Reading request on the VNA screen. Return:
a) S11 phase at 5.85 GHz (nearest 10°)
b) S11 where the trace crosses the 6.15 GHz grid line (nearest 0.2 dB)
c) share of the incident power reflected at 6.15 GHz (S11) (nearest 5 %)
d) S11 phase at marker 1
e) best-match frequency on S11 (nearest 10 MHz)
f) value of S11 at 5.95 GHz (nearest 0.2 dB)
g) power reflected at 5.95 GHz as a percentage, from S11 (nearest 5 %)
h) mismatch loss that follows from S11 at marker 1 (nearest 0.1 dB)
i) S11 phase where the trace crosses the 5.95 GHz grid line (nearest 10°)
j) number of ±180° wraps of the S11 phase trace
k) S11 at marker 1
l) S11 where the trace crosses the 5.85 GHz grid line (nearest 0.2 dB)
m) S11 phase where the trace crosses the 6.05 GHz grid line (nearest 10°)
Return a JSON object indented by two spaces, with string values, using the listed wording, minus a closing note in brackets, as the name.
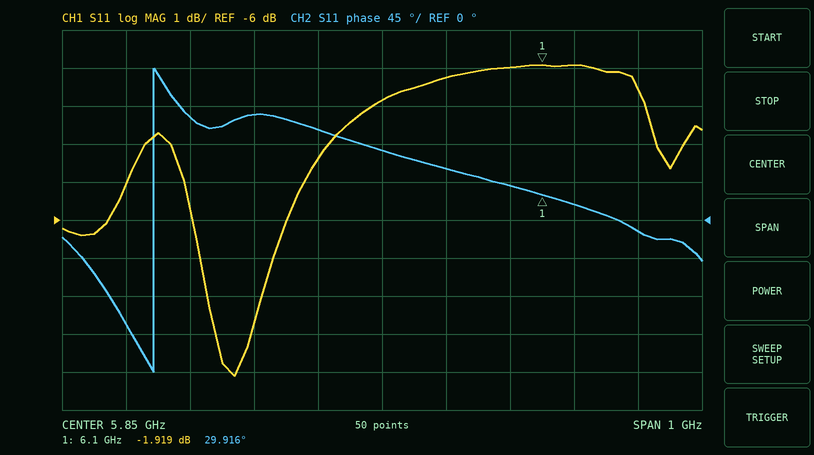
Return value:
{
  "S11 phase at 5.85 GHz": "80°",
  "S11 where the trace crosses the 6.15 GHz grid line": "-2.0 dB",
  "share of the incident power reflected at 6.15 GHz (S11)": "65 %",
  "S11 phase at marker 1": "29.916°",
  "best-match frequency on S11": "5.62 GHz",
  "value of S11 at 5.95 GHz": "-2.2 dB",
  "power reflected at 5.95 GHz as a percentage, from S11": "60 %",
  "mismatch loss that follows from S11 at marker 1": "4.5 dB",
  "S11 phase where the trace crosses the 5.95 GHz grid line": "60°",
  "number of ±180° wraps of the S11 phase trace": "1",
  "S11 at marker 1": "-1.919 dB",
  "S11 where the trace crosses the 5.85 GHz grid line": "-2.8 dB",
  "S11 phase where the trace crosses the 6.05 GHz grid line": "40°"
}
